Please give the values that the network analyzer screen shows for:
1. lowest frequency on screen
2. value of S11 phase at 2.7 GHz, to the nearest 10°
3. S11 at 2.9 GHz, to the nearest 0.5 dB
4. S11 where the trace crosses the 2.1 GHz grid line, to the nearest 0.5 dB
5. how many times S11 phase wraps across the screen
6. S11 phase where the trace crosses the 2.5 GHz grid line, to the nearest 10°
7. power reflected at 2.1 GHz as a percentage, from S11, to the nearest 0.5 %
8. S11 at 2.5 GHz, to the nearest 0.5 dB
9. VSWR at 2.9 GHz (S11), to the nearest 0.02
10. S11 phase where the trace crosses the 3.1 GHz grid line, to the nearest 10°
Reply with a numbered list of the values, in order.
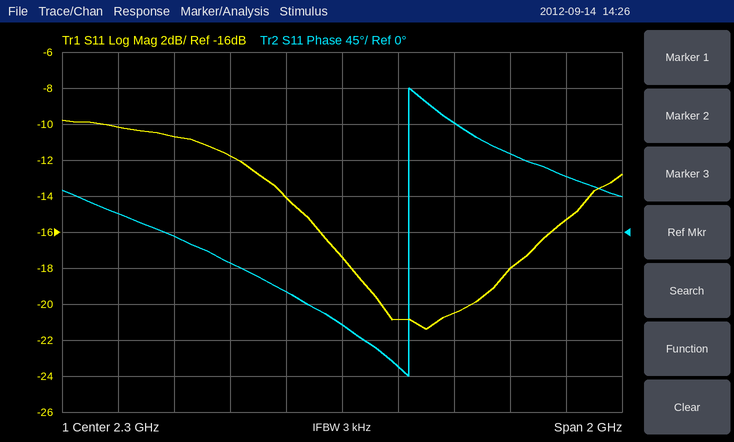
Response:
1. 1.3 GHz
2. 140°
3. -18.0 dB
4. -14.0 dB
5. 1
6. -170°
7. 4.0 %
8. -21.0 dB
9. 1.28
10. 70°
